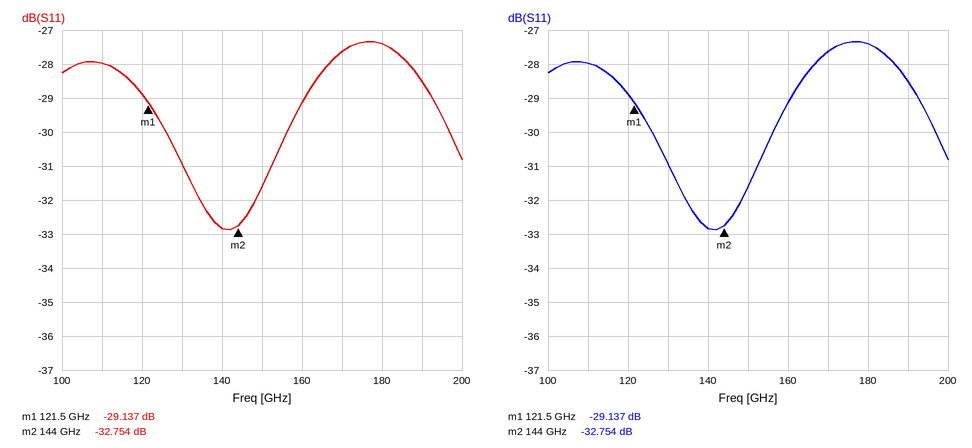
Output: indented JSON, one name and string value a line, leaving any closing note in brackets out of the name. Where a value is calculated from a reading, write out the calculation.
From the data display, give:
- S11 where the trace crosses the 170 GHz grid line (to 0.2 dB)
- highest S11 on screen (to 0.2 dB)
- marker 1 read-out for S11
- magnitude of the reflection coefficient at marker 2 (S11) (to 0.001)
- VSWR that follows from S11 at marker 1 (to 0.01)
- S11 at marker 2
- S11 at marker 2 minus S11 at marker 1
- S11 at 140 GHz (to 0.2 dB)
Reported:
{
  "S11 where the trace crosses the 170 GHz grid line": "-27.6 dB",
  "highest S11 on screen": "-27.4 dB",
  "marker 1 read-out for S11": "-29.137 dB",
  "magnitude of the reflection coefficient at marker 2 (S11)": "10^(-32.754/20) ≈ 0.023",
  "VSWR that follows from S11 at marker 1": "(1 + 0.0349)/(1 − 0.0349) ≈ 1.07",
  "S11 at marker 2": "-32.754 dB",
  "S11 at marker 2 minus S11 at marker 1": "-32.754 − (-29.137) = -3.617 dB",
  "S11 at 140 GHz": "-32.8 dB"
}
